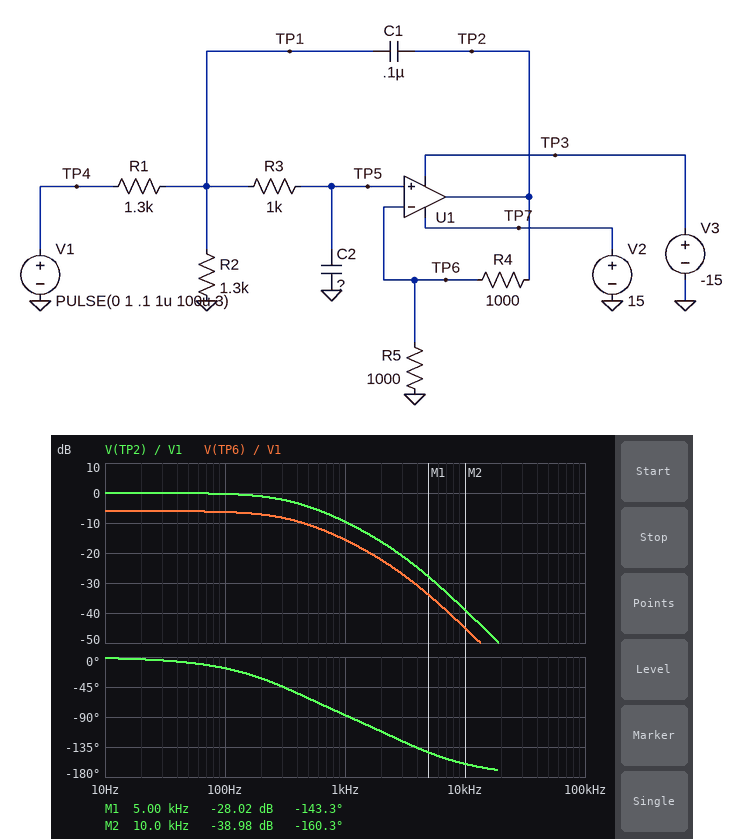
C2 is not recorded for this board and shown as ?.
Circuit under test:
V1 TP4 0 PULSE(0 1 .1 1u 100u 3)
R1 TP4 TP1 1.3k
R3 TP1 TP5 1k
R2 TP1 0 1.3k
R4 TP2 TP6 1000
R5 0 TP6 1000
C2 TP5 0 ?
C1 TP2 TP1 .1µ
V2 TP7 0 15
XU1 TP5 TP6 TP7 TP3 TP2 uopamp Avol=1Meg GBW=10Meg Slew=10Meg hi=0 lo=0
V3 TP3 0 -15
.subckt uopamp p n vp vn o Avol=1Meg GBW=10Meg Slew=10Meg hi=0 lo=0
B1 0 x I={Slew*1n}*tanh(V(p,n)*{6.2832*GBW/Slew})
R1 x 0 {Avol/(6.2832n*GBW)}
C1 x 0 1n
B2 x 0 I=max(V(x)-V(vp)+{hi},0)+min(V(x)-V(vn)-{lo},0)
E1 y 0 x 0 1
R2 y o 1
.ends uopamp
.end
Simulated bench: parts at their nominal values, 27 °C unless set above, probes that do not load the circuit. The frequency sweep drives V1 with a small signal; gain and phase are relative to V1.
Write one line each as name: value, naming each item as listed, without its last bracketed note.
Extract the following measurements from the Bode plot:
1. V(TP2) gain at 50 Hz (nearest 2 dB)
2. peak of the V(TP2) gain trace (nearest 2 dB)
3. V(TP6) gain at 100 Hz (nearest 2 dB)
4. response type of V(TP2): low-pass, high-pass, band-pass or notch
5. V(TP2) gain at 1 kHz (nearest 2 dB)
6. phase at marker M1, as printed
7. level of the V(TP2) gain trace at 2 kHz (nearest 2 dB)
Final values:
V(TP2) gain at 50 Hz: 0 dB
peak of the V(TP2) gain trace: 0 dB
V(TP6) gain at 100 Hz: -6 dB
response type of V(TP2): low-pass, high-pass, band-pass or notch: low-pass
V(TP2) gain at 1 kHz: -10 dB
phase at marker M1, as printed: -143.3 deg
level of the V(TP2) gain trace at 2 kHz: -16 dB
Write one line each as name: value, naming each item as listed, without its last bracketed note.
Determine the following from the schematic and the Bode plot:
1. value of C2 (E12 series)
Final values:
value of C2: 330 nF
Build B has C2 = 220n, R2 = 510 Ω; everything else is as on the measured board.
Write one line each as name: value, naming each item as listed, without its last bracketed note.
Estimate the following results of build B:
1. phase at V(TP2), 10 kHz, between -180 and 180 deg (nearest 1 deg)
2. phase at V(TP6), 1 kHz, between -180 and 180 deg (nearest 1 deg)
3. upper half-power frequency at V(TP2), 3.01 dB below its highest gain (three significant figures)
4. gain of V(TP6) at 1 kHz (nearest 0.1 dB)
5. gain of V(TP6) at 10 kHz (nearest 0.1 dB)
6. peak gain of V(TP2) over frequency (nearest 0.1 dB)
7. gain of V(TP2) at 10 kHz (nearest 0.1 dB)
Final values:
phase at V(TP2), 10 kHz, between -180 and 180 deg: -152 deg
phase at V(TP6), 1 kHz, between -180 and 180 deg: -68 deg
upper half-power frequency at V(TP2), 3.01 dB below its highest gain: 680 Hz
gain of V(TP6) at 1 kHz: -16.1 dB
gain of V(TP6) at 10 kHz: -41.9 dB
peak gain of V(TP2) over frequency: -5.0 dB
gain of V(TP2) at 10 kHz: -35.9 dB
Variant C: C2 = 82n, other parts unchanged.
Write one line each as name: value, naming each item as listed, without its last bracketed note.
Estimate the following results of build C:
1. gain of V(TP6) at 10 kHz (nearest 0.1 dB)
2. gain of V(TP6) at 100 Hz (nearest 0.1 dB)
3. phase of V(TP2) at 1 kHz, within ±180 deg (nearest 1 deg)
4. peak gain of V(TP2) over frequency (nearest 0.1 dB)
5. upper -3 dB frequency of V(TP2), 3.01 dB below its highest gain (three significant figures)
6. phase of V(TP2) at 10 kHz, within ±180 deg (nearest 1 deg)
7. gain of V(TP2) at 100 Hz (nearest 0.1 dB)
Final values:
gain of V(TP6) at 10 kHz: -32.3 dB
gain of V(TP6) at 100 Hz: -6.0 dB
phase of V(TP2) at 1 kHz, within ±180 deg: -29 deg
peak gain of V(TP2) over frequency: 1.5 dB
upper -3 dB frequency of V(TP2), 3.01 dB below its highest gain: 2.56 kHz
phase of V(TP2) at 10 kHz, within ±180 deg: -168 deg
gain of V(TP2) at 100 Hz: 0 dB
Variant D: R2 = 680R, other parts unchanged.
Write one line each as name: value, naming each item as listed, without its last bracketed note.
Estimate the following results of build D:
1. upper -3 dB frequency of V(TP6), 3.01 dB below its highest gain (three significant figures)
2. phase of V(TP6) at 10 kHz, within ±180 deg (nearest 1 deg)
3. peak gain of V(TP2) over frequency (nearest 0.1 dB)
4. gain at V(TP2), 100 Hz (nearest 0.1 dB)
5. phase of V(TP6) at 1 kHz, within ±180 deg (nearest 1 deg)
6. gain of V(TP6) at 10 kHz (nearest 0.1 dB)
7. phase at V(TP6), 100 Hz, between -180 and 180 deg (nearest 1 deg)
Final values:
upper -3 dB frequency of V(TP6), 3.01 dB below its highest gain: 399 Hz
phase of V(TP6) at 10 kHz, within ±180 deg: -155 deg
peak gain of V(TP2) over frequency: -3.3 dB
gain at V(TP2), 100 Hz: -3.5 dB
phase of V(TP6) at 1 kHz, within ±180 deg: -81 deg
gain of V(TP6) at 10 kHz: -45.3 dB
phase at V(TP6), 100 Hz, between -180 and 180 deg: -15 deg
